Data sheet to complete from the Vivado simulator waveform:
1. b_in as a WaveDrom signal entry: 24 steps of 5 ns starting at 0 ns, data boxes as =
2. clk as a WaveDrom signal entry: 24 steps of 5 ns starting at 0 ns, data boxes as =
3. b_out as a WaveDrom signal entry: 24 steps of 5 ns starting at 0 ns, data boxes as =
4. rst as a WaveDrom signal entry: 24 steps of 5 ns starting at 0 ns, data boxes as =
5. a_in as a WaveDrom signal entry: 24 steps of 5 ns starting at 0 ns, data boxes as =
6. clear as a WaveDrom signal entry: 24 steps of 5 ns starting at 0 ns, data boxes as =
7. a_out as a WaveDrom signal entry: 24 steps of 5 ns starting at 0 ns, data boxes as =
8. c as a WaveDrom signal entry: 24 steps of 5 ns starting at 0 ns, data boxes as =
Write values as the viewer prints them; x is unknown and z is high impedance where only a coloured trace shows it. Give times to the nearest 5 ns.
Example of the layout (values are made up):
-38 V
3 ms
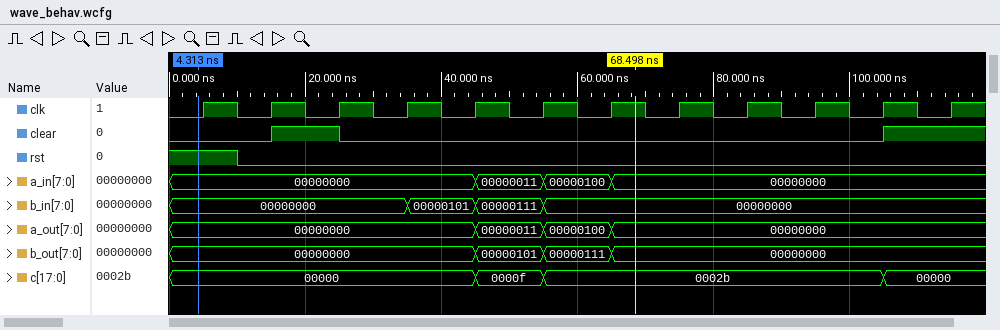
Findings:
{name: 'b_in', wave: '=......=.=.=............', data: '00000000 00000101 00000111 00000000'}
{name: 'clk', wave: '010101010101010101010101'}
{name: 'b_out', wave: '=........=.=.=..........', data: '00000000 00000101 00000111 00000000'}
{name: 'rst', wave: '1.0.....................'}
{name: 'a_in', wave: '=........=.=.=..........', data: '00000000 00000011 00000100 00000000'}
{name: 'clear', wave: '0..1.0...............1..'}
{name: 'a_out', wave: '=........=.=.=..........', data: '00000000 00000011 00000100 00000000'}
{name: 'c', wave: '=........=.=.........=..', data: '00000 0000f 0002b 00000'}
